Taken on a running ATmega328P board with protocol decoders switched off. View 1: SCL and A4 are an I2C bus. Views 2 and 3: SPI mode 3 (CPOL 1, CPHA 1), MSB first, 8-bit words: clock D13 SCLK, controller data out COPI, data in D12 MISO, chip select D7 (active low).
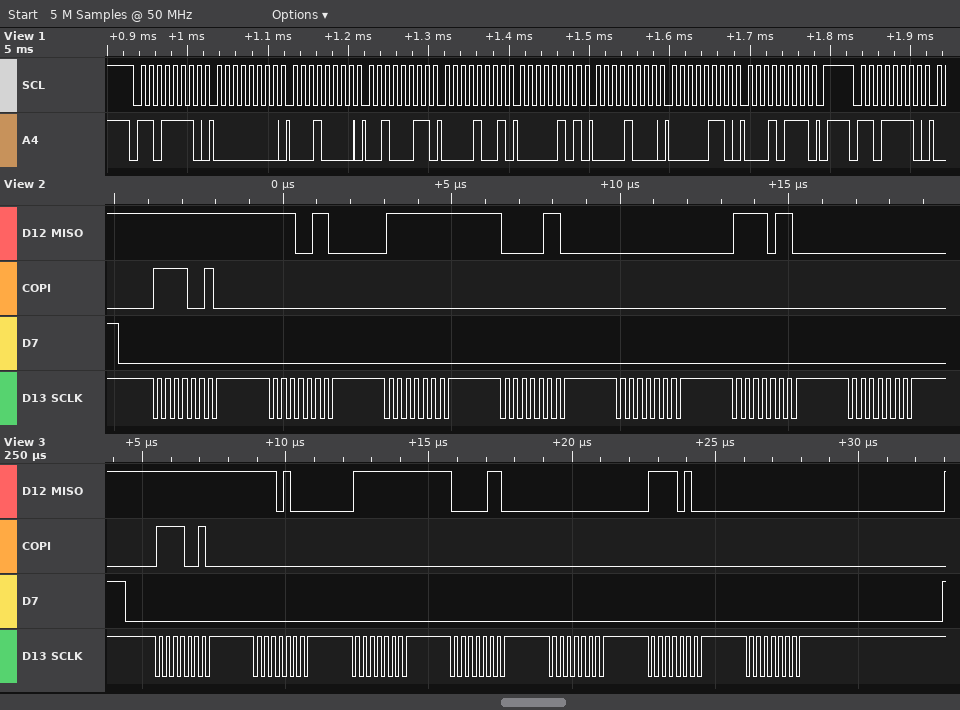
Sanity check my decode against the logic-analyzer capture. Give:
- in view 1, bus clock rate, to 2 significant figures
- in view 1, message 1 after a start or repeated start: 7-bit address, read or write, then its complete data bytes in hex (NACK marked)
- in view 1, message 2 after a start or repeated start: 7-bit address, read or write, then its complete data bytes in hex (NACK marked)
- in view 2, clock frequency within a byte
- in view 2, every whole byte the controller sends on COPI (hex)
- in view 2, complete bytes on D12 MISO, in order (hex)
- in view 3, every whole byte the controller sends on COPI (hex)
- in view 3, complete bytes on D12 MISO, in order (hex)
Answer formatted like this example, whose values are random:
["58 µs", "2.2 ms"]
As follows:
["100 kHz", "0x6F write: 00 10 23 09 05 08 06 17", "0x6F write", "4 MHz", "F2 00 00 00 00 00 00", "FF E6 FF 06 00 F6 00", "F2 00 00 00 00 00 00", "FF E8 FF 06 00 F4 00"]
